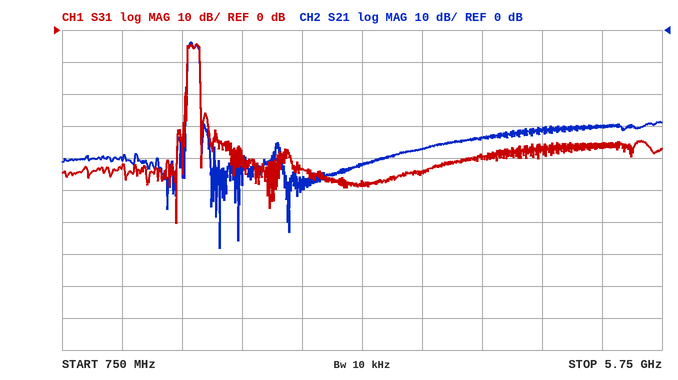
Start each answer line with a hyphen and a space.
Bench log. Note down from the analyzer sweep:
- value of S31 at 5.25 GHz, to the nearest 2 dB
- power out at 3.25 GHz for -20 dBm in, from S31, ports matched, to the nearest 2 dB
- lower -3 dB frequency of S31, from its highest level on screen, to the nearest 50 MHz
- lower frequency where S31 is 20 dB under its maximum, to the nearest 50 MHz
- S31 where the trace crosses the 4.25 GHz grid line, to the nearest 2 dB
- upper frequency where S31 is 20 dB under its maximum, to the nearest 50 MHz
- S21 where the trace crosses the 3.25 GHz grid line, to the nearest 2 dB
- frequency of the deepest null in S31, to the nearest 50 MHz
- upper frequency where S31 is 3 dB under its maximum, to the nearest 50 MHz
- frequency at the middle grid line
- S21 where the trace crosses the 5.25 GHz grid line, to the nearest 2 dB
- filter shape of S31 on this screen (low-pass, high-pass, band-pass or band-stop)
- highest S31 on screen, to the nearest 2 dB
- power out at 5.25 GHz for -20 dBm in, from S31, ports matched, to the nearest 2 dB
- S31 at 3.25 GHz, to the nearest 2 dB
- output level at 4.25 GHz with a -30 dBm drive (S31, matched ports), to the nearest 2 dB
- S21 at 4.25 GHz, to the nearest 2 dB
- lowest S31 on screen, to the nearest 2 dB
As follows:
- -36 dB
- -68 dBm
- 1.80 GHz
- 1.80 GHz
- -40 dB
- 1.90 GHz
- -42 dB
- 1.70 GHz
- 1.90 GHz
- 3.25 GHz
- -30 dB
- band-pass
- -4 dB
- -56 dBm
- -48 dB
- -70 dBm
- -34 dB
- -60 dB
